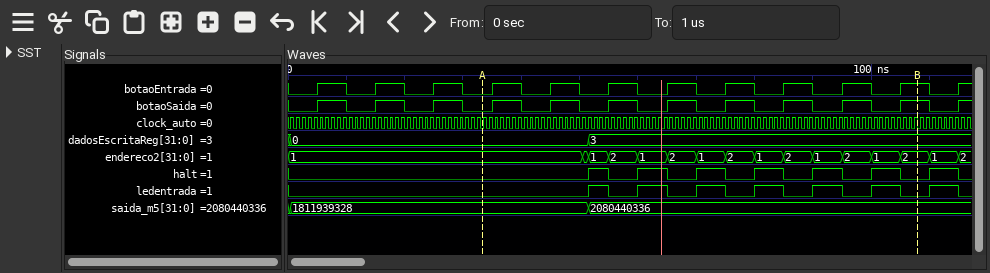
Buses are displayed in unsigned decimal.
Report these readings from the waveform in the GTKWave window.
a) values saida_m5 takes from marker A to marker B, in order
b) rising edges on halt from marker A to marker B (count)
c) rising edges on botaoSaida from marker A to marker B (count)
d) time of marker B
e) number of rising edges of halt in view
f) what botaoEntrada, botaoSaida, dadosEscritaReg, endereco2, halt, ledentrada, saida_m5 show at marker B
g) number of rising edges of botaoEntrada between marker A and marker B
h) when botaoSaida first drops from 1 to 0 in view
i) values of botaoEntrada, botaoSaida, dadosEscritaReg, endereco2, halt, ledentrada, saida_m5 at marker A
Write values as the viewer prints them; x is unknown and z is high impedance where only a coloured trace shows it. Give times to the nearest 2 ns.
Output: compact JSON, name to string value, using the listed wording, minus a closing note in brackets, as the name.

{"values saida_m5 takes from marker A to marker B, in order": "1811939328, 2080440336", "rising edges on halt from marker A to marker B": "6", "rising edges on botaoSaida from marker A to marker B": "8", "time of marker B": "108 ns", "number of rising edges of halt in view": "7", "what botaoEntrada, botaoSaida, dadosEscritaReg, endereco2, halt, ledentrada, saida_m5 show at marker B": "botaoEntrada=1, botaoSaida=1, dadosEscritaReg=3, endereco2=2, halt=0, ledentrada=0, saida_m5=2080440336", "number of rising edges of botaoEntrada between marker A and marker B": "8", "when botaoSaida first drops from 1 to 0 in view": "10 ns", "values of botaoEntrada, botaoSaida, dadosEscritaReg, endereco2, halt, ledentrada, saida_m5 at marker A": "botaoEntrada=0, botaoSaida=0, dadosEscritaReg=0, endereco2=1, halt=0, ledentrada=0, saida_m5=1811939328"}
